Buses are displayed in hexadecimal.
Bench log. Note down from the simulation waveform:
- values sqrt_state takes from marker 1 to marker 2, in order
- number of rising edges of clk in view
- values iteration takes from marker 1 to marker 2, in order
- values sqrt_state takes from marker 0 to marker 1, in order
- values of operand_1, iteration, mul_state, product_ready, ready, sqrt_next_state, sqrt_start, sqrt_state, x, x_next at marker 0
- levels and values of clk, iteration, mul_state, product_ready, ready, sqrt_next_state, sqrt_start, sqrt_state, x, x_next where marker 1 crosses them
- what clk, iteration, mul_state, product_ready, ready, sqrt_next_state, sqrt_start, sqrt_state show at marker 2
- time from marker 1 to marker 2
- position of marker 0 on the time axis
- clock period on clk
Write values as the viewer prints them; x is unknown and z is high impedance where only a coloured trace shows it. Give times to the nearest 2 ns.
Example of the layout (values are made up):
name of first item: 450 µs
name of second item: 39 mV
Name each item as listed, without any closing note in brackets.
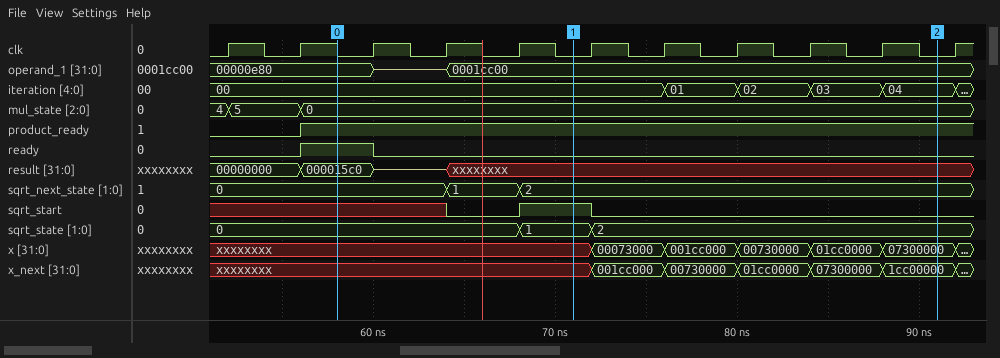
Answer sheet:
values sqrt_state takes from marker 1 to marker 2, in order: 1, 2
number of rising edges of clk in view: 11
values iteration takes from marker 1 to marker 2, in order: 00, 01, 02, 03, 04
values sqrt_state takes from marker 0 to marker 1, in order: 0, 1
values of operand_1, iteration, mul_state, product_ready, ready, sqrt_next_state, sqrt_start, sqrt_state, x, x_next at marker 0: operand_1=00000e80, iteration=00, mul_state=0, product_ready=1, ready=1, sqrt_next_state=0, sqrt_start=x, sqrt_state=0, x=xxxxxxxx, x_next=xxxxxxxx
levels and values of clk, iteration, mul_state, product_ready, ready, sqrt_next_state, sqrt_start, sqrt_state, x, x_next where marker 1 crosses them: clk=0, iteration=00, mul_state=0, product_ready=1, ready=0, sqrt_next_state=2, sqrt_start=1, sqrt_state=1, x=xxxxxxxx, x_next=xxxxxxxx
what clk, iteration, mul_state, product_ready, ready, sqrt_next_state, sqrt_start, sqrt_state show at marker 2: clk=0, iteration=04, mul_state=0, product_ready=1, ready=0, sqrt_next_state=2, sqrt_start=0, sqrt_state=2
time from marker 1 to marker 2: 20 ns
position of marker 0 on the time axis: 58 ns
clock period on clk: 4 ns
